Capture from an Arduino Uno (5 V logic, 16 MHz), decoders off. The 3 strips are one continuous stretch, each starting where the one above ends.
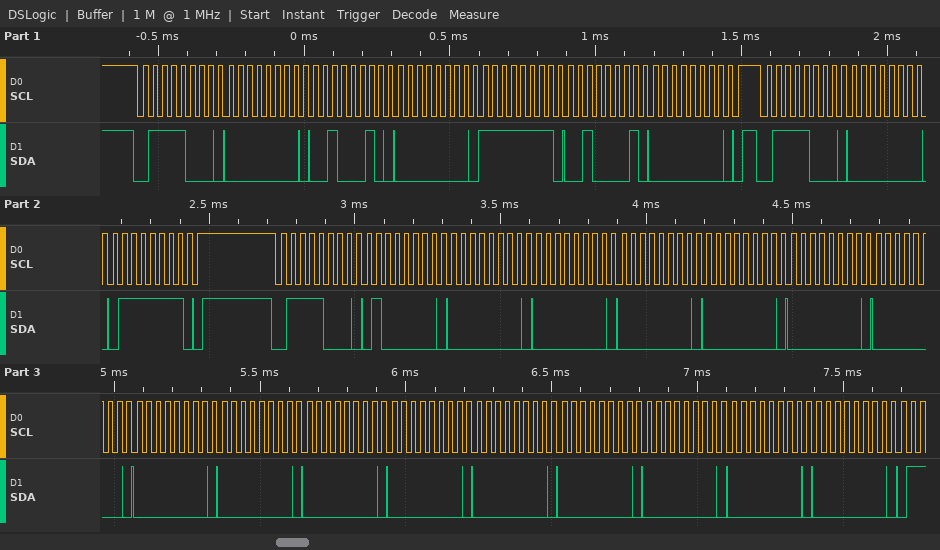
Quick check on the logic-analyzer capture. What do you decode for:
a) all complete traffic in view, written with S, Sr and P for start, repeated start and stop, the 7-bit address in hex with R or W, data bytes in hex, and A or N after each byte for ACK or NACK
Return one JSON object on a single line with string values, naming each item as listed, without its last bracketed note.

{"all complete traffic in view, written with S, Sr and P for start, repeated start and stop, the 7-bit address in hex with R or W, data bytes in hex, and A or N after each byte for ACK or NACK": "S 3CW A 00 A 22 A 00 A FF A 21 A 00 A P S 3CW A 00 A 7F A P S 3CW A 40 A 00 A 00 A 00 A 00 A 00 A 00 A 00 A 00 A 00 A 00 A 00 A 00 A 00 A 00 A 00 A"}
